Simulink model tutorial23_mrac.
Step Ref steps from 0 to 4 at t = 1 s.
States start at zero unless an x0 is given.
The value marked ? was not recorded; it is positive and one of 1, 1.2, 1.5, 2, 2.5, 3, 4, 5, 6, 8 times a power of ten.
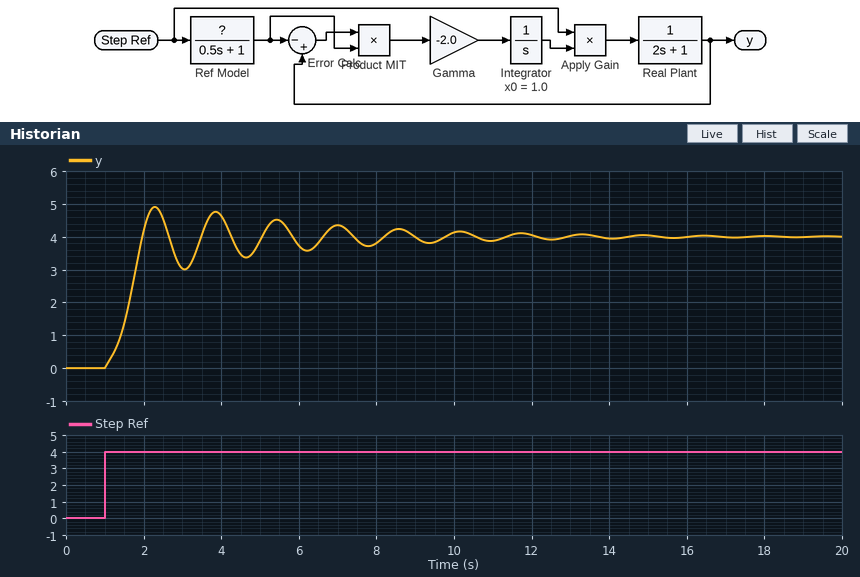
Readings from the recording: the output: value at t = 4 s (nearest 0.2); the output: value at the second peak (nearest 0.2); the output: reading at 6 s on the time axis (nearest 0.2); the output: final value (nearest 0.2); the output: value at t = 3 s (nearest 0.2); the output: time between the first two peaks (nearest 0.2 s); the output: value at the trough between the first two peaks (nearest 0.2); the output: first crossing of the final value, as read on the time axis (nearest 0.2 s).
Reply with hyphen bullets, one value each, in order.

- 4.6
- 4.8
- 3.8
- 4.0
- 3.0
- 1.6 s
- 3.0
- 2.0 s
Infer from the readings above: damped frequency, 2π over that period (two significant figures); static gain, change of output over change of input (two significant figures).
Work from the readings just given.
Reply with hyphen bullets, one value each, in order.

- 3.9 rad/s
- 1.0
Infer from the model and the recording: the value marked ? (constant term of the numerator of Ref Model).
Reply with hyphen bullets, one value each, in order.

- 1
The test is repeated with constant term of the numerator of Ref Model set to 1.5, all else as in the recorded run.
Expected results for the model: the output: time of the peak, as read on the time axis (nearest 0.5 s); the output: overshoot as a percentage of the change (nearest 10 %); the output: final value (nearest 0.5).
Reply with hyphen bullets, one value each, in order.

- 2.0 s
- 20 %
- 6.0
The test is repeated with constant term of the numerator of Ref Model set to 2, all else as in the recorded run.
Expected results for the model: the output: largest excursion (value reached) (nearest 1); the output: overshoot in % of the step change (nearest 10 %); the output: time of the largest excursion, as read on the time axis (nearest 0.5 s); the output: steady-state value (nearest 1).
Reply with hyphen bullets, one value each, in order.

- 10
- 20 %
- 3.0 s
- 8
